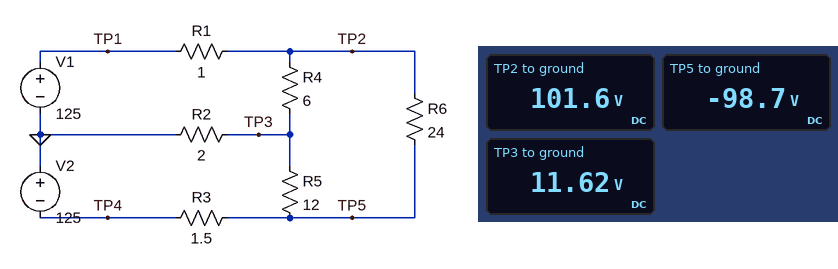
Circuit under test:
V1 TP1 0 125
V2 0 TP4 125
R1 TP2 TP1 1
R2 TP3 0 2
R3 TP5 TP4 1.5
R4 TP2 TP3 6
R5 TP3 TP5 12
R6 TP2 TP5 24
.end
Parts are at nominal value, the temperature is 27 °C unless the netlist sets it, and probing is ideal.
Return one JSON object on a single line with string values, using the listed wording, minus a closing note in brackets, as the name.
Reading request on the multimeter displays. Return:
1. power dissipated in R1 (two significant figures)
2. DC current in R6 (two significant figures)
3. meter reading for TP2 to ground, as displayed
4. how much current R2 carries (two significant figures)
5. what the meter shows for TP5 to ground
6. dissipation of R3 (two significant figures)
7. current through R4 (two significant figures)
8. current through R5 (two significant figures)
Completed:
{"power dissipated in R1": "550 W", "DC current in R6": "8.3 A", "meter reading for TP2 to ground, as displayed": "101.6 V", "how much current R2 carries": "5.8 A", "what the meter shows for TP5 to ground": "-98.7 V", "dissipation of R3": "460 W", "current through R4": "15 A", "current through R5": "9.2 A"}
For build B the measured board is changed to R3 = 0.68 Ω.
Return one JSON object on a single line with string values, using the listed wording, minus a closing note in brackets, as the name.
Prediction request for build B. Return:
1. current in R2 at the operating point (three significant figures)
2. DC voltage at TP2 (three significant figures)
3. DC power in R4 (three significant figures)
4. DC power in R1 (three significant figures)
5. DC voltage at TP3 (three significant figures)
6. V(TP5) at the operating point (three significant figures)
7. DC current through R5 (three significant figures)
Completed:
{"current in R2 at the operating point": "4.99 A", "DC voltage at TP2": "101 V", "DC power in R4": "1.38 kW", "DC power in R1": "578 W", "DC voltage at TP3": "9.99 V", "V(TP5) at the operating point": "-112 V", "DC current through R5": "10.2 A"}
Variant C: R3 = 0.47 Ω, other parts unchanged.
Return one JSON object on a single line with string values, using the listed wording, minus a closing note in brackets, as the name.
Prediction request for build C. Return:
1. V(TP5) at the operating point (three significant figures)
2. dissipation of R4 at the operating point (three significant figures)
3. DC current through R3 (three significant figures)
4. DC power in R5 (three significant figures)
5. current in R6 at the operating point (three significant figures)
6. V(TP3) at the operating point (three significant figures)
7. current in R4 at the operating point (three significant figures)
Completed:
{"V(TP5) at the operating point": "-116 V", "dissipation of R4 at the operating point": "1.39 kW", "DC current through R3": "19.5 A", "DC power in R5": "1.31 kW", "current in R6 at the operating point": "9.03 A", "V(TP3) at the operating point": "9.52 V", "current in R4 at the operating point": "15.2 A"}
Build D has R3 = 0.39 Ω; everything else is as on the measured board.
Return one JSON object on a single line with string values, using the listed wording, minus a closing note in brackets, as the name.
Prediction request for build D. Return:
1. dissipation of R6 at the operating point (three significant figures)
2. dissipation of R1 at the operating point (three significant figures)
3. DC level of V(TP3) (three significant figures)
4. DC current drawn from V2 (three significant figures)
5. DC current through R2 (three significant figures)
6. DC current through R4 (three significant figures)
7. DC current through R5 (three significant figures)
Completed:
{"dissipation of R6 at the operating point": "1.98 kW", "dissipation of R1 at the operating point": "591 W", "DC level of V(TP3)": "9.34 V", "DC current drawn from V2": "19.6 A", "DC current through R2": "4.67 A", "DC current through R4": "15.2 A", "DC current through R5": "10.6 A"}
